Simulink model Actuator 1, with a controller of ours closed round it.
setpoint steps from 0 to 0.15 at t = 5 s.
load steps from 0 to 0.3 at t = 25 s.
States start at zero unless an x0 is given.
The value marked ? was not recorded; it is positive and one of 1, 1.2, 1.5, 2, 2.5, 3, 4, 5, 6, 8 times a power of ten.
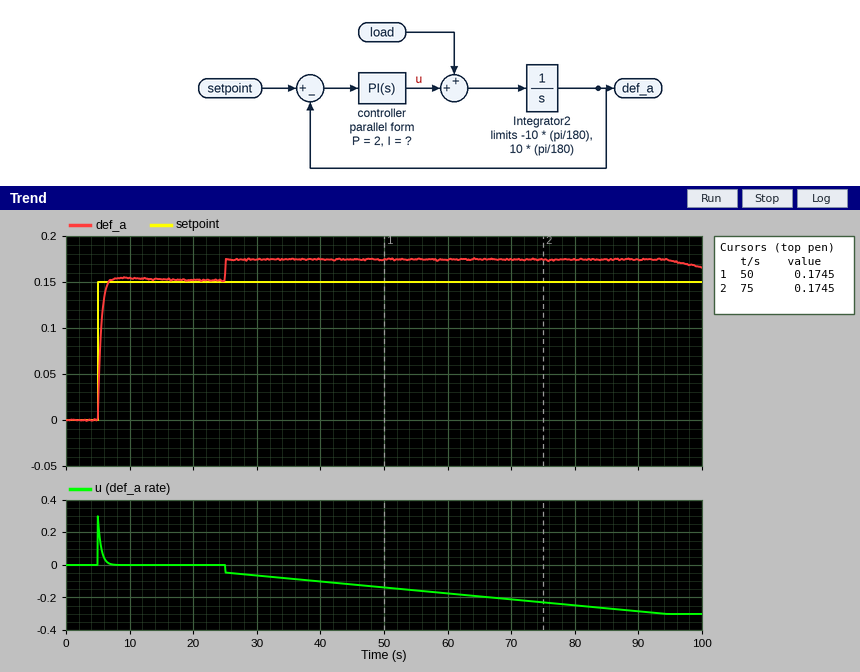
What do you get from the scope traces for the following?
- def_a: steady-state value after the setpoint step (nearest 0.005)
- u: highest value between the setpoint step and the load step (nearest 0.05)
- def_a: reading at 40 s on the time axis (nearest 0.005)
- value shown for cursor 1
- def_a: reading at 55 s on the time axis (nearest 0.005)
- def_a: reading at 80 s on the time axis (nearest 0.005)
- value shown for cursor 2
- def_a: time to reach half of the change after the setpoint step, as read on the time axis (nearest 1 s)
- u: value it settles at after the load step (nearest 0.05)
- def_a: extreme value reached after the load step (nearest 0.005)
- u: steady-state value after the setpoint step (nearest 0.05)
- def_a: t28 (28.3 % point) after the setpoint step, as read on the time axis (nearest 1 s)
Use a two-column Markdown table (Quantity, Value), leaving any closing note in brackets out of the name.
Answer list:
| Quantity | Value |
|---|---|
| def_a: steady-state value after the setpoint step | 0.150 |
| u: highest value between the setpoint step and the load step | 0.30 |
| def_a: reading at 40 s on the time axis | 0.175 |
| value shown for cursor 1 | 0.1745 |
| def_a: reading at 55 s on the time axis | 0.175 |
| def_a: reading at 80 s on the time axis | 0.175 |
| value shown for cursor 2 | 0.1745 |
| def_a: time to reach half of the change after the setpoint step, as read on the time axis | 5 s |
| u: value it settles at after the load step | -0.30 |
| def_a: extreme value reached after the load step | 0.175 |
| u: steady-state value after the setpoint step | 0.00 |
| def_a: t28 (28.3 % point) after the setpoint step, as read on the time axis | 5 s |
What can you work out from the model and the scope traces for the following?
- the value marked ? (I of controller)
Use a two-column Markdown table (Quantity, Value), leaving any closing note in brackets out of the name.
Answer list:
| Quantity | Value |
|---|---|
| the value marked ? | 0.15 |
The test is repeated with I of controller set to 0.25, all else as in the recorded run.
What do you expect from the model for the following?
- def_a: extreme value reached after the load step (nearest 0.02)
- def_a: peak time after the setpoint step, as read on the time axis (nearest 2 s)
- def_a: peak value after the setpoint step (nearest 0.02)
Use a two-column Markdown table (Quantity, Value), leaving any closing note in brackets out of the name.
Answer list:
| Quantity | Value |
|---|---|
| def_a: extreme value reached after the load step | 0.18 |
| def_a: peak time after the setpoint step, as read on the time axis | 8 s |
| def_a: peak value after the setpoint step | 0.16 |
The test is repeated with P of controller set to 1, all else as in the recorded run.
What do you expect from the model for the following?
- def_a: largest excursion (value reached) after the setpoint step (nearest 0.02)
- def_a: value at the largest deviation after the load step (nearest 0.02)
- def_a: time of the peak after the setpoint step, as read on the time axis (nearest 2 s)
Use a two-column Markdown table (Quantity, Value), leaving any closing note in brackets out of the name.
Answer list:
| Quantity | Value |
|---|---|
| def_a: largest excursion (value reached) after the setpoint step | 0.16 |
| def_a: value at the largest deviation after the load step | 0.18 |
| def_a: time of the peak after the setpoint step, as read on the time axis | 10 s |
